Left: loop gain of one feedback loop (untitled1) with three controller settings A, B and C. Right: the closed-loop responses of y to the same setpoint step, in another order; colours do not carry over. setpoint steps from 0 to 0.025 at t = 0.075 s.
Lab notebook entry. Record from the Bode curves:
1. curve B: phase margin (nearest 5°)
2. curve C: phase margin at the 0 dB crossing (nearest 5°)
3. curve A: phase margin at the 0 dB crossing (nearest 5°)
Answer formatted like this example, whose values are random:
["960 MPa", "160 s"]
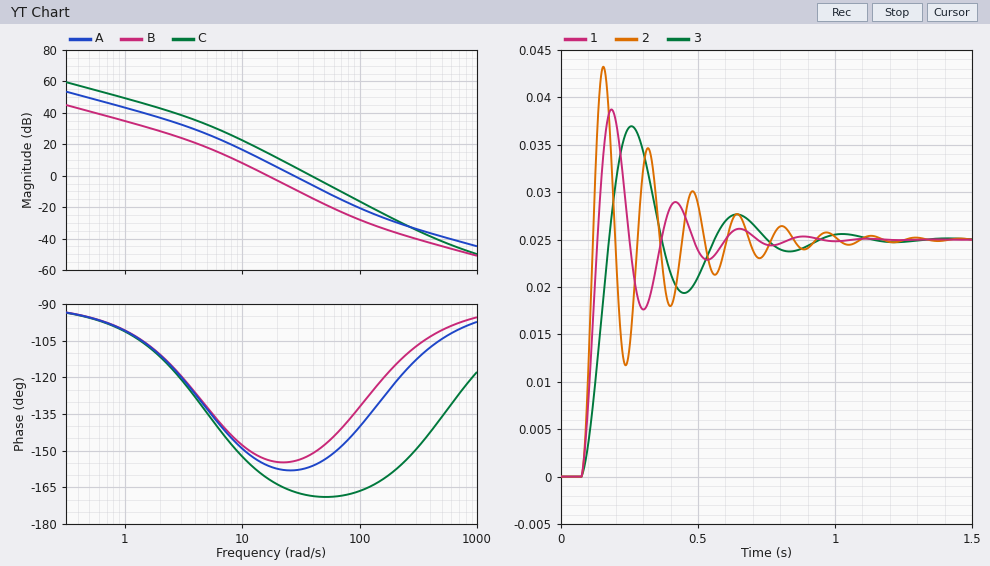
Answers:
["25°", "10°", "20°"]
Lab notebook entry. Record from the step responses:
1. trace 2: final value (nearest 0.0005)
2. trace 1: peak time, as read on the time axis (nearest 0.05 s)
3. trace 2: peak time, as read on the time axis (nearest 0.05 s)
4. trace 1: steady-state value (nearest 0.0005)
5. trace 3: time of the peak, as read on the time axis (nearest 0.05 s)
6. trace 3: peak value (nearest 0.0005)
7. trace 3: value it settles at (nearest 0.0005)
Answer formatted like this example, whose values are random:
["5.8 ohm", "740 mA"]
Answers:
["0.0250", "0.20 s", "0.15 s", "0.0250", "0.25 s", "0.0370", "0.0250"]
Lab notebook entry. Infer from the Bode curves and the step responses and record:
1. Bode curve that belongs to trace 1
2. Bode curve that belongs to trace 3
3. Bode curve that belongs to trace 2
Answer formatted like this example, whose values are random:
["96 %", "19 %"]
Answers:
["A", "B", "C"]
